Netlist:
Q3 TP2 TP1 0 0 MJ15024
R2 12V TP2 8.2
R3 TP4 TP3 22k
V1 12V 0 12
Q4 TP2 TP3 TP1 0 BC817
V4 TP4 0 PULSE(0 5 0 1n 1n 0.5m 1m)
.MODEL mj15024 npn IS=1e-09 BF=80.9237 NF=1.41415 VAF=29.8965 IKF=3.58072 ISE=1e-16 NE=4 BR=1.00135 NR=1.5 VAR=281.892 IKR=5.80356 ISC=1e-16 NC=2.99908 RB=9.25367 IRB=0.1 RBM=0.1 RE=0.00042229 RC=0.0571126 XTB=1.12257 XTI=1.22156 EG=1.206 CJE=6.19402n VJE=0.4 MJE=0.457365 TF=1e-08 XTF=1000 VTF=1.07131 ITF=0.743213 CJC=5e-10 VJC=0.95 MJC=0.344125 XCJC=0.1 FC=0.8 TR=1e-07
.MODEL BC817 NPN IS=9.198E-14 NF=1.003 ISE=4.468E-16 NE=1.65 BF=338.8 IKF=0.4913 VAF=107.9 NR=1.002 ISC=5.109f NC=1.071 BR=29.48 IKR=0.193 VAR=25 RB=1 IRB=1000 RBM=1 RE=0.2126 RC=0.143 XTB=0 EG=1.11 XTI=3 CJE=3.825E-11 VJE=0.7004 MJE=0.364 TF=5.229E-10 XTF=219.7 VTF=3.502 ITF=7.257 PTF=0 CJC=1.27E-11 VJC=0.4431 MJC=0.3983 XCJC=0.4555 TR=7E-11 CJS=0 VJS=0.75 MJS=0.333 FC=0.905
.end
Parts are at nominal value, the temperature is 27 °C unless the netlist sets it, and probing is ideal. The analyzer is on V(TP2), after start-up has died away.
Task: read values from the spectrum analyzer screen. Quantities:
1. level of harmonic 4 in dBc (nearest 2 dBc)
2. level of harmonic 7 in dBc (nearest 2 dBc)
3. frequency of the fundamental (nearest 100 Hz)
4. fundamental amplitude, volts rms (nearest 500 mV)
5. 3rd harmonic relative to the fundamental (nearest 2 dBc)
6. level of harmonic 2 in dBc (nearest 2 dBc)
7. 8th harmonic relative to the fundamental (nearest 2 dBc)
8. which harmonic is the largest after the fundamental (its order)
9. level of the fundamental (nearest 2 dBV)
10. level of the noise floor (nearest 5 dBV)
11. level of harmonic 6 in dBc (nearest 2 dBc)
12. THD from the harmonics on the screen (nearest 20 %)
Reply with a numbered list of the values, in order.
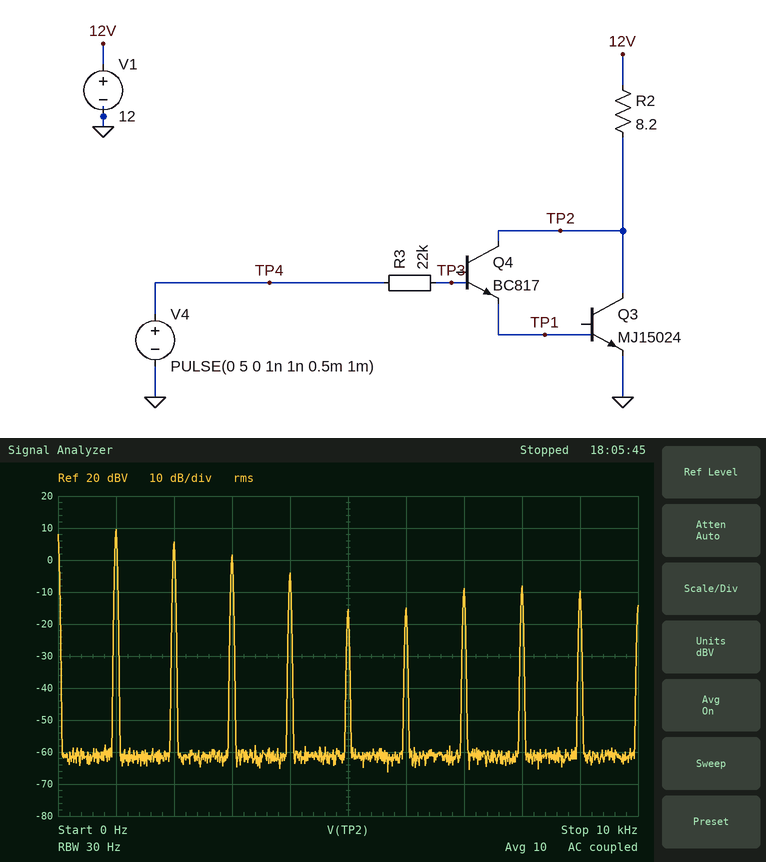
1. -14 dBc
2. -18 dBc
3. 1.0 kHz
4. 3.0 V
5. -8 dBc
6. -4 dBc
7. -18 dBc
8. 2
9. 10 dBV
10. -60 dBV
11. -24 dBc
12. 80 %
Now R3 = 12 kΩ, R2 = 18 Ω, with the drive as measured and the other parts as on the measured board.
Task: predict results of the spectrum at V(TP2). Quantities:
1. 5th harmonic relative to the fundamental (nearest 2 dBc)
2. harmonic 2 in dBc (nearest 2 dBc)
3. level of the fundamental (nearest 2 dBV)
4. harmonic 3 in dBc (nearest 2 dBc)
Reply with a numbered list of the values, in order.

1. -14 dBc
2. -6 dBc
3. 12 dBV
4. -26 dBc
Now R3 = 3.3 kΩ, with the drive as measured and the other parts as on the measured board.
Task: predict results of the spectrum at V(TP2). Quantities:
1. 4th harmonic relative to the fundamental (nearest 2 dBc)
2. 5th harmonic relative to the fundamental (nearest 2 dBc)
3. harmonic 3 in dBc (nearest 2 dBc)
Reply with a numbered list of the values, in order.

1. -10 dBc
2. -18 dBc
3. -6 dBc
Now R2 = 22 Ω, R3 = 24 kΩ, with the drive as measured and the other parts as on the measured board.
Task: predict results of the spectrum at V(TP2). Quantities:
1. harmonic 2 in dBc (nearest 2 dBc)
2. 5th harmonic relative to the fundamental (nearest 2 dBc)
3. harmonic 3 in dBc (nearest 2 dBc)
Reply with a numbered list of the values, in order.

1. -8 dBc
2. -18 dBc
3. -20 dBc
